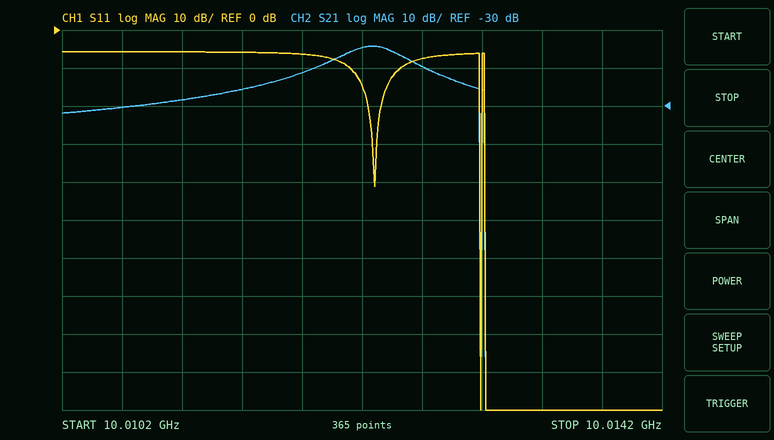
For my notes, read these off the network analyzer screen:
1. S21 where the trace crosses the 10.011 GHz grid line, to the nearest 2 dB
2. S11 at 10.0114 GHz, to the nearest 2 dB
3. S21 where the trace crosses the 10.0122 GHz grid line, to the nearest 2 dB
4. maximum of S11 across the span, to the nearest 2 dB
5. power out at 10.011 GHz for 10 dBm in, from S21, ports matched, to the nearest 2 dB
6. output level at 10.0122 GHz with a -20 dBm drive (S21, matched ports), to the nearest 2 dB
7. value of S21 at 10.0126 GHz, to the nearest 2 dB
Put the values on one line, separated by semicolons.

-28 dB; -6 dB; -14 dB; -6 dB; -18 dBm; -34 dBm; -20 dB
